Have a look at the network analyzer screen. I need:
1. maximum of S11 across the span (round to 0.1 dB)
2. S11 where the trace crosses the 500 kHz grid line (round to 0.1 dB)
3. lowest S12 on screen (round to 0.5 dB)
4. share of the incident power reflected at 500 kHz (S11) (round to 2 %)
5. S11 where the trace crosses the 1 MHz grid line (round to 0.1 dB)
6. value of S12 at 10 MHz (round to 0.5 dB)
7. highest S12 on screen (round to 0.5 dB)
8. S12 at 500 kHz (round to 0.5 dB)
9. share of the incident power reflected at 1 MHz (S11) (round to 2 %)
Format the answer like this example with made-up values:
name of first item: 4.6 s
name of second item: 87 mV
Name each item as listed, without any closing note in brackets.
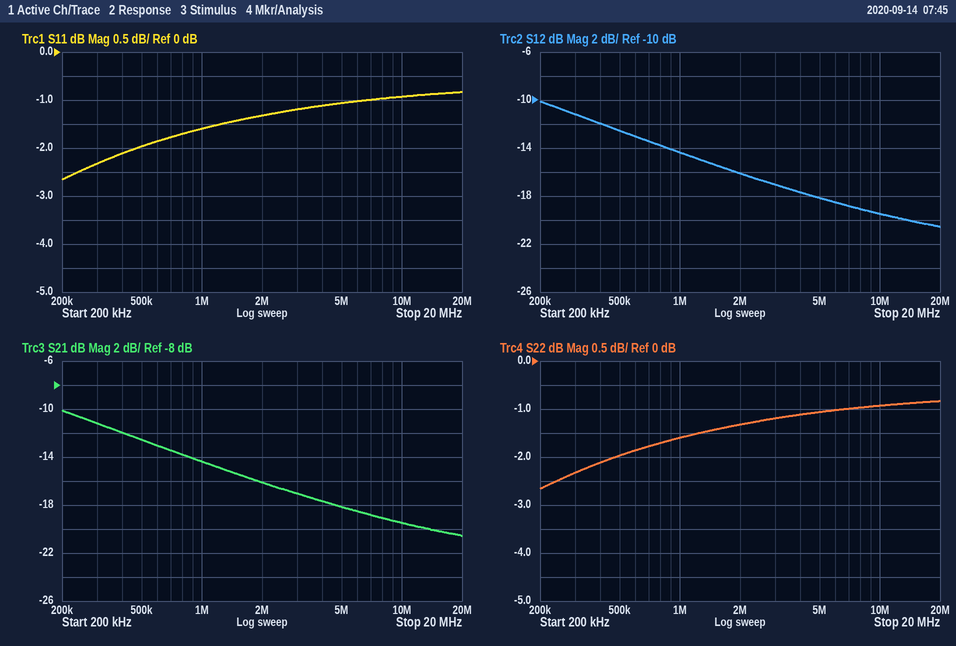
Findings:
maximum of S11 across the span: -0.8 dB
S11 where the trace crosses the 500 kHz grid line: -2.0 dB
lowest S12 on screen: -20.5 dB
share of the incident power reflected at 500 kHz (S11): 64 %
S11 where the trace crosses the 1 MHz grid line: -1.6 dB
value of S12 at 10 MHz: -19.5 dB
highest S12 on screen: -10.0 dB
S12 at 500 kHz: -12.5 dB
share of the incident power reflected at 1 MHz (S11): 70 %
